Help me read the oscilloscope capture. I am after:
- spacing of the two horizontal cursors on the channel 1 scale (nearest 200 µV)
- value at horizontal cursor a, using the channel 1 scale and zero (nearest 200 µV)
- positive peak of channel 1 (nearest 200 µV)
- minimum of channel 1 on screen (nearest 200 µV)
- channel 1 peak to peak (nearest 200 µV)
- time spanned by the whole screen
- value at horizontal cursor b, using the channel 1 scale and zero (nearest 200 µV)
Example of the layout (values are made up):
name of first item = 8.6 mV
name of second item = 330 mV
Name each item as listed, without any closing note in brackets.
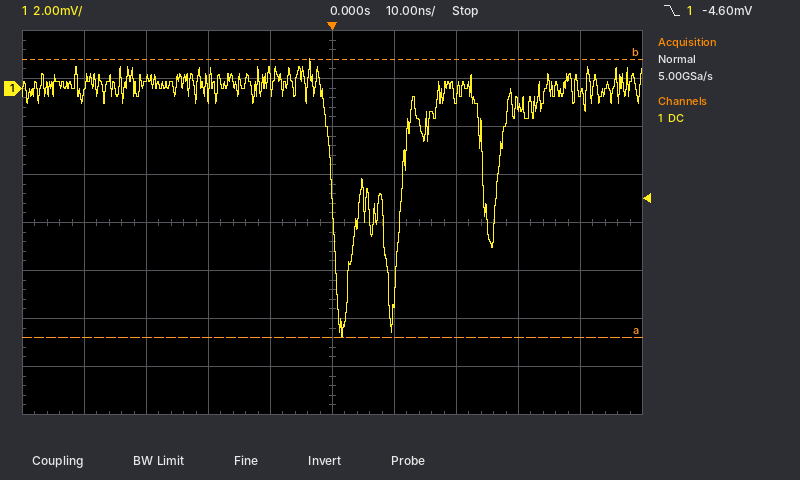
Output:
spacing of the two horizontal cursors on the channel 1 scale = 11.6 mV
value at horizontal cursor a, using the channel 1 scale and zero = -10.4 mV
positive peak of channel 1 = 1.2 mV
minimum of channel 1 on screen = -10.4 mV
channel 1 peak to peak = 11.6 mV
time spanned by the whole screen = 100 ns
value at horizontal cursor b, using the channel 1 scale and zero = 1.2 mV
